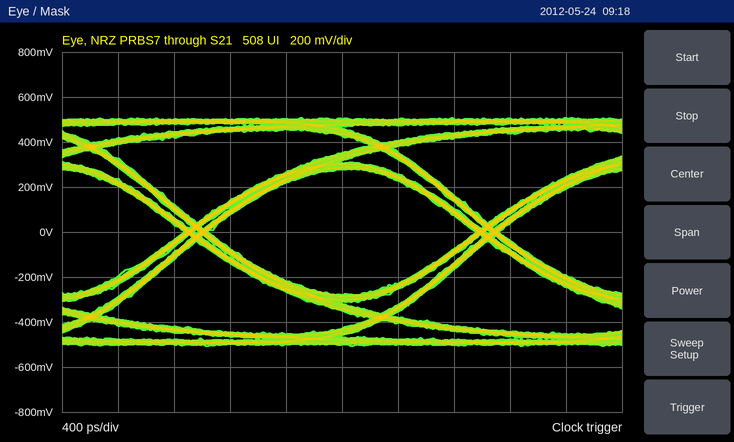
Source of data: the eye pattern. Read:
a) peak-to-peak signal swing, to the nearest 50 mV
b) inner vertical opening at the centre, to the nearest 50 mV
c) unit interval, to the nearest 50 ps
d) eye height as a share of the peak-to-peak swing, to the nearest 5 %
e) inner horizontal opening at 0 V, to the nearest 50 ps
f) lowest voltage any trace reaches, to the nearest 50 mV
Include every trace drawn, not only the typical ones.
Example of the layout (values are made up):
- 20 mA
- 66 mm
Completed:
- 1.00 V
- 550 mV
- 2.10 ns
- 55 %
- 1.90 ns
- -500 mV
